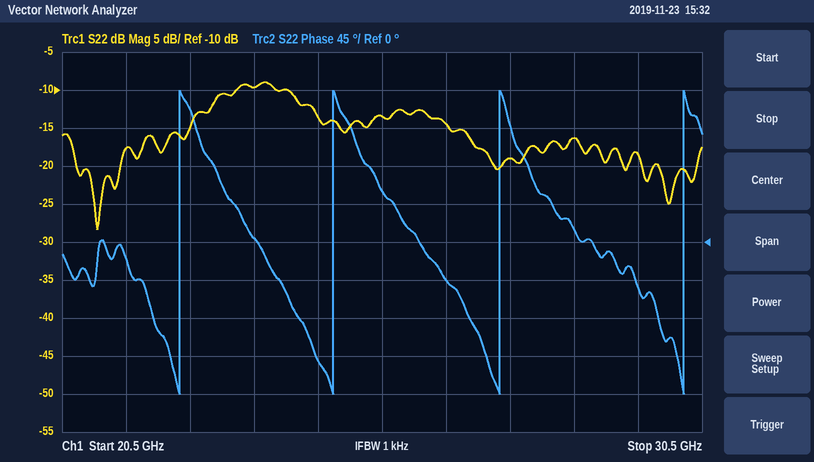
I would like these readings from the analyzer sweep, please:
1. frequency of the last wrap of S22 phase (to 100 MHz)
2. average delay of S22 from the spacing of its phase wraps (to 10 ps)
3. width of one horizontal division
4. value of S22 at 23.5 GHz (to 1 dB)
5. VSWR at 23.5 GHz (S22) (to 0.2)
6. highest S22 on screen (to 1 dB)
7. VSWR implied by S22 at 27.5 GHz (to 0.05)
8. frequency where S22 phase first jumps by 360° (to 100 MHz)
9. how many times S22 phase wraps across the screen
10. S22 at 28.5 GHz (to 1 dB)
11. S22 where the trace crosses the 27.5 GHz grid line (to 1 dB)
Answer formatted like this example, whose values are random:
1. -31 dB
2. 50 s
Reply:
1. 30.2 GHz
2. 380 ps
3. 1 GHz
4. -10 dB
5. 2.0
6. -9 dB
7. 1.25
8. 22.3 GHz
9. 4
10. -16 dB
11. -19 dB
